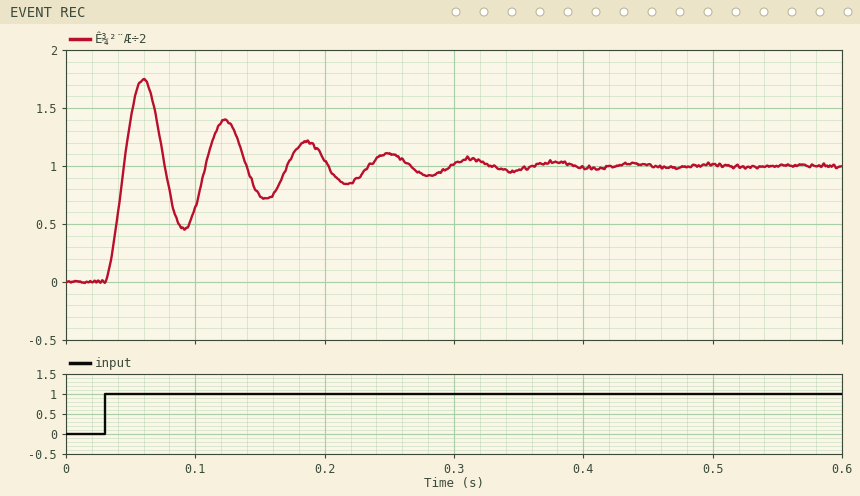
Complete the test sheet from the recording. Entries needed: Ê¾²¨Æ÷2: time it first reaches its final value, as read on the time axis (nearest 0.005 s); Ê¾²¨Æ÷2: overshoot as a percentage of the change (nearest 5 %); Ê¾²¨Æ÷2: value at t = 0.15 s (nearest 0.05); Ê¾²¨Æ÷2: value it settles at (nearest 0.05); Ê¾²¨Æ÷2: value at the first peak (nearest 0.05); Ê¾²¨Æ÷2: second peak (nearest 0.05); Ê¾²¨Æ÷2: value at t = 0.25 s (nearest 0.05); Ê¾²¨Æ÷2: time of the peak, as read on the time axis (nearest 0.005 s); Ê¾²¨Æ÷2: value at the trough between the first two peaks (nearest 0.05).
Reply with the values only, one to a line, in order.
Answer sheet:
0.045 s
75 %
0.75
1.00
1.75
1.40
1.10
0.060 s
0.45
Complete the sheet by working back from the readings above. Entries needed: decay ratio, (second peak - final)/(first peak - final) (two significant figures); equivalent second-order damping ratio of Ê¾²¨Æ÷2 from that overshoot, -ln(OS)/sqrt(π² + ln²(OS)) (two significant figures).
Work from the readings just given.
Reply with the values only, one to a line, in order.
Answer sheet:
0.53
0.091
